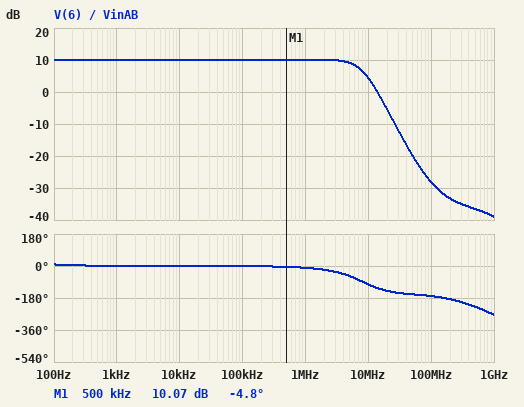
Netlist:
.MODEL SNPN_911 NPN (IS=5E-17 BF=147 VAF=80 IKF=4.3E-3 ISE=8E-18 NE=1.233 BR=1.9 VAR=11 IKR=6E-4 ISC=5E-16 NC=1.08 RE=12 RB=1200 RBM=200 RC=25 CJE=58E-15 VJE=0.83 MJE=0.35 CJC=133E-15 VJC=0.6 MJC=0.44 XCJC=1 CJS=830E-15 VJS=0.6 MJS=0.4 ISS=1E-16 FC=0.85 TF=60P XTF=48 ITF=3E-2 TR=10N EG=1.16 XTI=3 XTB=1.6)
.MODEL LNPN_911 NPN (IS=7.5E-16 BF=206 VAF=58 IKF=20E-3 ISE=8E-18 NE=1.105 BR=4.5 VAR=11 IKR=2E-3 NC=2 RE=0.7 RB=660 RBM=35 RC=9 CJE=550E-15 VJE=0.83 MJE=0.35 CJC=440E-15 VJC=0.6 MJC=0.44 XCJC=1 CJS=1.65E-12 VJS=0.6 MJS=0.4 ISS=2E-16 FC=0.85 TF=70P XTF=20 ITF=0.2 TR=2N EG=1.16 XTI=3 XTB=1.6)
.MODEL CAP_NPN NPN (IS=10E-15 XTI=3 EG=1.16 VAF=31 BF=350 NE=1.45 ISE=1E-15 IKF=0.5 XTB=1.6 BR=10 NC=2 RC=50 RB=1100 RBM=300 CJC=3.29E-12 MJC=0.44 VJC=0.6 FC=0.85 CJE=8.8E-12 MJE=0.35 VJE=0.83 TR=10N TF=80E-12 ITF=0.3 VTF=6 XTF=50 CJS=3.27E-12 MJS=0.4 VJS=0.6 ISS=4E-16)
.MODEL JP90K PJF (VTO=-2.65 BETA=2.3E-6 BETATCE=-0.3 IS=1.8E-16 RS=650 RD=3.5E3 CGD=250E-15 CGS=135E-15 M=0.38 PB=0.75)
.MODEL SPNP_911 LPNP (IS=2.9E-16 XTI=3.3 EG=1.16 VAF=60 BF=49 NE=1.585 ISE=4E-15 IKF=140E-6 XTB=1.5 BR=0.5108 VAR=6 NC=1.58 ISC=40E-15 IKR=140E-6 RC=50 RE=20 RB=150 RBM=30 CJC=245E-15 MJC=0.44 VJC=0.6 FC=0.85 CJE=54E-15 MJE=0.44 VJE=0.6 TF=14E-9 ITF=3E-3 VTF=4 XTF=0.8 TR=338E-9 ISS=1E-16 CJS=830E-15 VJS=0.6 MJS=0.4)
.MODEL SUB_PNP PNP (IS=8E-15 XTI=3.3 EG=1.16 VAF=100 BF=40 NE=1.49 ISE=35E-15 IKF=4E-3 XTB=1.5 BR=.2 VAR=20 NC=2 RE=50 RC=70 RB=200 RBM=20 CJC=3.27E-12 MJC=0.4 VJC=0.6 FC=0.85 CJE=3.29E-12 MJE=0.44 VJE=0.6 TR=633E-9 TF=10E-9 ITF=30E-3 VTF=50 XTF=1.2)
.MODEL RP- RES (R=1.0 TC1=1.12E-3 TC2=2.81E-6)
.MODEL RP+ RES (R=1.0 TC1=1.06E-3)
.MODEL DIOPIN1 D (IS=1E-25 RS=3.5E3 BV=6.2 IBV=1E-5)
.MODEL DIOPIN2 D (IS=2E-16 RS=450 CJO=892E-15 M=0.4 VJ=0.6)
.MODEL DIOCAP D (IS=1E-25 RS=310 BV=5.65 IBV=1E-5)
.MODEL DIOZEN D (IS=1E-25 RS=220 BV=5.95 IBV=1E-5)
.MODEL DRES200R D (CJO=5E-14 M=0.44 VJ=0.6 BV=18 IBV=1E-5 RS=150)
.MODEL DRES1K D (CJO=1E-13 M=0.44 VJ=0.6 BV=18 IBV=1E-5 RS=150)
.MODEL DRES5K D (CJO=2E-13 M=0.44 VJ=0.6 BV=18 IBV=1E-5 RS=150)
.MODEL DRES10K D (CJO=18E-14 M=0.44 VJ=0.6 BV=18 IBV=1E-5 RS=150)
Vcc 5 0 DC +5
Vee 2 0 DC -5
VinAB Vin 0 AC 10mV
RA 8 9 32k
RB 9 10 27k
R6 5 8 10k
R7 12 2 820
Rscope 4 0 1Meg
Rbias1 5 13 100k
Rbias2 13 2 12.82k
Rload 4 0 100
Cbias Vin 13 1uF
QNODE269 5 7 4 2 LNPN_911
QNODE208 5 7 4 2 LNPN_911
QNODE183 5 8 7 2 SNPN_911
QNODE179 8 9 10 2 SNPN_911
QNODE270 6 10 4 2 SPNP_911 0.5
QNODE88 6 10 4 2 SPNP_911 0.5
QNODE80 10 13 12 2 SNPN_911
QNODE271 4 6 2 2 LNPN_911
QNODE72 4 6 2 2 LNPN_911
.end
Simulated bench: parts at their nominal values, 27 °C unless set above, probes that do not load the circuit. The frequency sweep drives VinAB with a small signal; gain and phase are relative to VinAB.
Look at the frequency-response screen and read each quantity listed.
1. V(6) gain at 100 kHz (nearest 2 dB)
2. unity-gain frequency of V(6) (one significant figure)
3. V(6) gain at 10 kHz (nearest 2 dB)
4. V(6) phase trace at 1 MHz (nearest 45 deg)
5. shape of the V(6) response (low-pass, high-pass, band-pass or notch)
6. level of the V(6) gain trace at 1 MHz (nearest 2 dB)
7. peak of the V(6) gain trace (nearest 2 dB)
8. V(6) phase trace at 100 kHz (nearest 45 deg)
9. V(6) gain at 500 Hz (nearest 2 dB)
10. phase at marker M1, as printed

10 dB
10 MHz
10 dB
0 deg
low-pass
10 dB
10 dB
0 deg
10 dB
-4.8 deg
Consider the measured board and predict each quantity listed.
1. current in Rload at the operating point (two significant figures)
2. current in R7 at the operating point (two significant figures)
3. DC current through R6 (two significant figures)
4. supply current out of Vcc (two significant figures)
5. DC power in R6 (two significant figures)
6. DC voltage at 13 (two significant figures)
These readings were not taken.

670 µA
390 µA
390 µA
510 µA
1.5 mW
-3.9 V
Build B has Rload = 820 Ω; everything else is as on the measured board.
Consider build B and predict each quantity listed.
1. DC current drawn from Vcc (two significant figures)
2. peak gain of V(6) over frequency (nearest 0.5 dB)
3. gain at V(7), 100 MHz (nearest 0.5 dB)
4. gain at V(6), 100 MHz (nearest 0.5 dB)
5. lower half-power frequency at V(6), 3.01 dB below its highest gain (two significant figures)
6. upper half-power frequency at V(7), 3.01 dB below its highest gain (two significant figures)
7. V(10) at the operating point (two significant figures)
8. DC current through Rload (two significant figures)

540 µA
4.0 dB
-21.5 dB
-25.5 dB
18 Hz
6.1 MHz
-670 mV
120 µA
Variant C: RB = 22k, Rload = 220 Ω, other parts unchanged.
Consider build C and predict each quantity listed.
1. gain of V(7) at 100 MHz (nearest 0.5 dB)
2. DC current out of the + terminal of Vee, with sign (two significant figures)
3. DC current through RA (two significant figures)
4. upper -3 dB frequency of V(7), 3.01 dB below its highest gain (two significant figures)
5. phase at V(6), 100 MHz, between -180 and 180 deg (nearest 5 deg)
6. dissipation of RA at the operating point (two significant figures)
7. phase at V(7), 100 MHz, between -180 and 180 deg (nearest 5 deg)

-21.0 dB
-2.5 mA
38 µA
11 MHz
-135 deg
47 µW
15 deg
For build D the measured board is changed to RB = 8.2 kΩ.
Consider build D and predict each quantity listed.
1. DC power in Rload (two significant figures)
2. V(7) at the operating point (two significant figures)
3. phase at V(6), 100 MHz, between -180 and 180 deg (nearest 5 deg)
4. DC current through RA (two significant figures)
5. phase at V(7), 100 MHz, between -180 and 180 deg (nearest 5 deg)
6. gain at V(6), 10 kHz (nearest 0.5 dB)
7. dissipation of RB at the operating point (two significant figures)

42 mW
3.2 V
-105 deg
71 µA
165 deg
-9.0 dB
41 µW
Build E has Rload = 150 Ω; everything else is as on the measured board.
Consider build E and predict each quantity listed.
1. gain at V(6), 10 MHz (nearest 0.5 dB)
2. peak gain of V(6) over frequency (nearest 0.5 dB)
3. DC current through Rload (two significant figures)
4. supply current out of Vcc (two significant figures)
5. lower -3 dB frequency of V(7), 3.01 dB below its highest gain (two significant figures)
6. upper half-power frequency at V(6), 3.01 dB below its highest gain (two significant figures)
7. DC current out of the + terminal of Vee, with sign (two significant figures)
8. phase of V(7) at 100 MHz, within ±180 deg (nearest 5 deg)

4.0 dB
9.0 dB
500 µA
520 µA
16 Hz
7.8 MHz
-1.0 mA
150 deg
